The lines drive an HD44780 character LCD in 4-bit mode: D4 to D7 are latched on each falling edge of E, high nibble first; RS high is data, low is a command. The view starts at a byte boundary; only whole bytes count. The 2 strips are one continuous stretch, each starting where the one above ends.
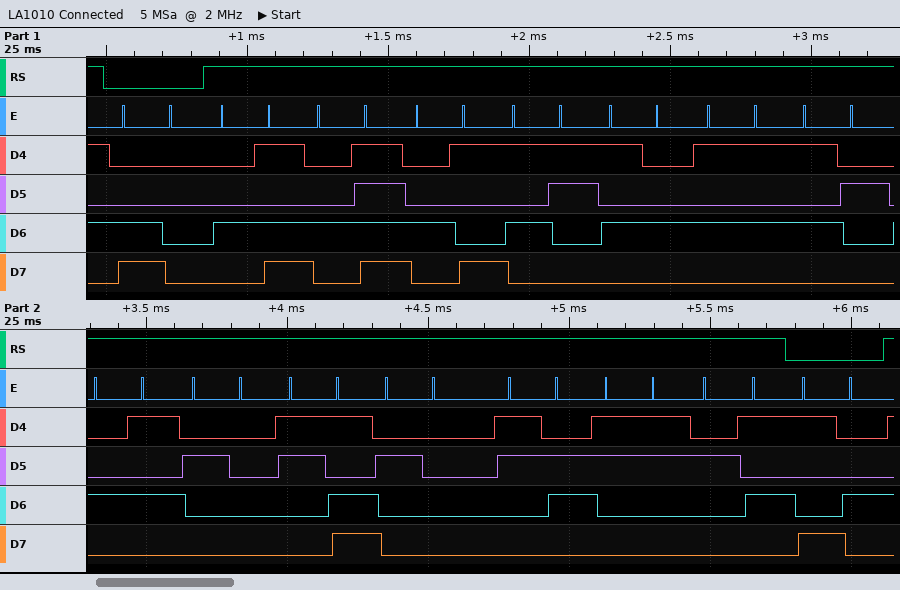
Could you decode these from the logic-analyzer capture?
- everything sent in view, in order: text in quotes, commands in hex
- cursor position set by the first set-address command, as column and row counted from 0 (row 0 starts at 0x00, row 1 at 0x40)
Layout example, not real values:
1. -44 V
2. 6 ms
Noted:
1. 0xC0 "MOISTURE = 63%" 0x94
2. column 0, row 1
